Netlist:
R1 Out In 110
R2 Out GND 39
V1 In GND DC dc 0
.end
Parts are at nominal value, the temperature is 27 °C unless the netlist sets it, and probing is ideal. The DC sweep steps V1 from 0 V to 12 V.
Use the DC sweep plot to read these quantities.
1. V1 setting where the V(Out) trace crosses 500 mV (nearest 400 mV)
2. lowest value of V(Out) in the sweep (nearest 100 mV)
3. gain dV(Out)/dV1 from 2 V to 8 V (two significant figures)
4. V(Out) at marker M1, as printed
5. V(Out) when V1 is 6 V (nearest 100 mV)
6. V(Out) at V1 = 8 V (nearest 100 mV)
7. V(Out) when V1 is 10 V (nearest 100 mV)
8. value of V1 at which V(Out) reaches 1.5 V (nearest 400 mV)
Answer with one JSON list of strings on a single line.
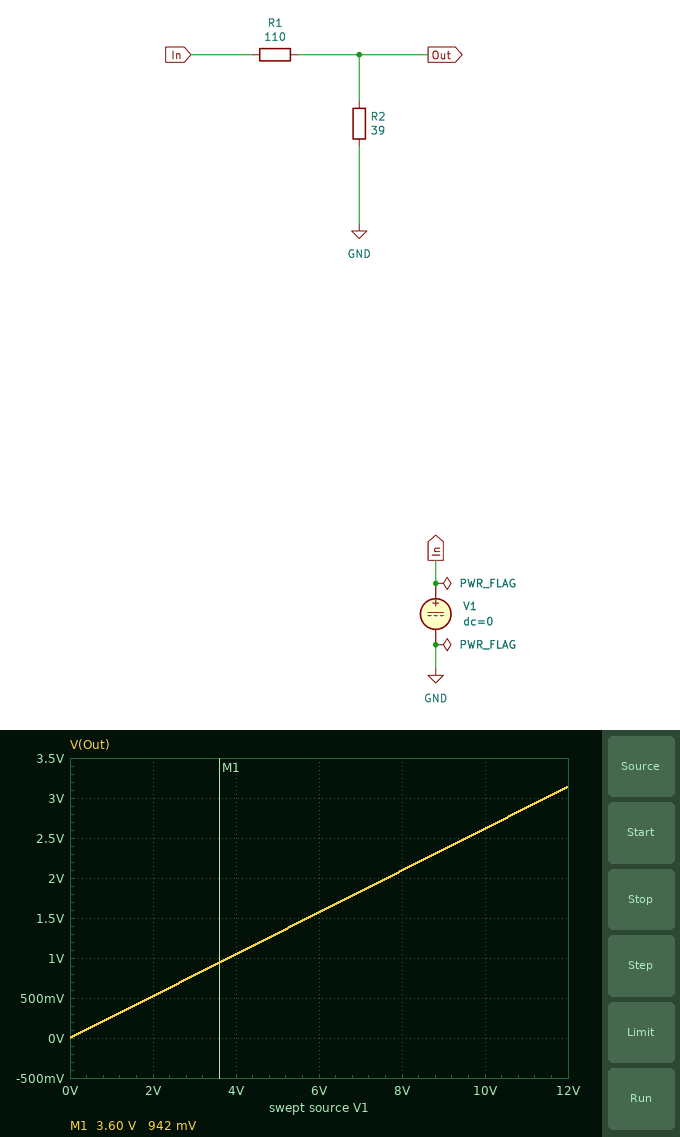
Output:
["2.0 V", "0 V", "0.26 V/V", "942 mV", "1.6 V", "2.1 V", "2.6 V", "5.6 V"]
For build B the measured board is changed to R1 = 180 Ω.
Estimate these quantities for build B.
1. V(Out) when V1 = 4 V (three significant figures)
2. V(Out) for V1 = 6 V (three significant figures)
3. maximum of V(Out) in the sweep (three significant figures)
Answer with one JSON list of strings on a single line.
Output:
["712 mV", "1.07 V", "2.14 V"]
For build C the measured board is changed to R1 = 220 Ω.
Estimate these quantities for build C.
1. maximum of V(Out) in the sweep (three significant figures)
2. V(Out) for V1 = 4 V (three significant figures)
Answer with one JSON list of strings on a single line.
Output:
["1.81 V", "602 mV"]
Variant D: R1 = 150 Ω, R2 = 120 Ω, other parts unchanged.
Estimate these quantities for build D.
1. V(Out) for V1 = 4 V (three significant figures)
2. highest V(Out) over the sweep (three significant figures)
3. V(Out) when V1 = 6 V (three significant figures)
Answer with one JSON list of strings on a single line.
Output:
["1.78 V", "5.33 V", "2.67 V"]
